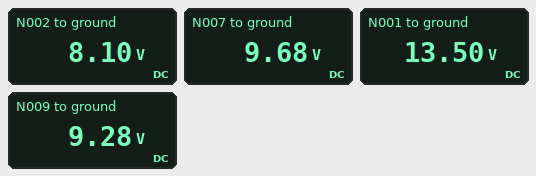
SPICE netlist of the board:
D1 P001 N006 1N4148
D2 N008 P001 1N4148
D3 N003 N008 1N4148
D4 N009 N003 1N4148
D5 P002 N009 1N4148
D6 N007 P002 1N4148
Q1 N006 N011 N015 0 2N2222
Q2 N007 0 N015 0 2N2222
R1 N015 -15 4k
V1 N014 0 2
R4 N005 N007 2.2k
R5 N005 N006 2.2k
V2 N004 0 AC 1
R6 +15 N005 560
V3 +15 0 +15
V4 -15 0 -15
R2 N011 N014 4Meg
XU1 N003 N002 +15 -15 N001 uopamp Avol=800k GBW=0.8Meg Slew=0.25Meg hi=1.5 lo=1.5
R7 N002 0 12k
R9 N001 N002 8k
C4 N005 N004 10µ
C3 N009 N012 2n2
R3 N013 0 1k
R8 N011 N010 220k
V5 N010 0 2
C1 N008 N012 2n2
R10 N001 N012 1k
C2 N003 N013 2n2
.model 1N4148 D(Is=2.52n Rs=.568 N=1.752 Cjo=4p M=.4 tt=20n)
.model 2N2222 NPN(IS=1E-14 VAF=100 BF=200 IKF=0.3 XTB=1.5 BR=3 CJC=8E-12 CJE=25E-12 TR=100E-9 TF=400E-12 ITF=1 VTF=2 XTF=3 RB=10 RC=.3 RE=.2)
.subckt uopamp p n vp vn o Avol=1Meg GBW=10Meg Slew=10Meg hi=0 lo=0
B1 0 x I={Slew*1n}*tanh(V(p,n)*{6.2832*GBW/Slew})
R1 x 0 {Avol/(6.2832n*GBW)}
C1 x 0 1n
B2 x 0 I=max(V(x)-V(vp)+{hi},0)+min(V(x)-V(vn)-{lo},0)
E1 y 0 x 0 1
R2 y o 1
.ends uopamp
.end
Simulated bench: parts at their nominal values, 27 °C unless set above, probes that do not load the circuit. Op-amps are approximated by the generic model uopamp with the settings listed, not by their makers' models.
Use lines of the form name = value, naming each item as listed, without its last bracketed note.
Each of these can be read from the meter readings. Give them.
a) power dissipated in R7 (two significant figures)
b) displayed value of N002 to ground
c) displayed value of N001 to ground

power dissipated in R7 = 5.5 mW
displayed value of N002 to ground = 8.10 V
displayed value of N001 to ground = 13.50 V
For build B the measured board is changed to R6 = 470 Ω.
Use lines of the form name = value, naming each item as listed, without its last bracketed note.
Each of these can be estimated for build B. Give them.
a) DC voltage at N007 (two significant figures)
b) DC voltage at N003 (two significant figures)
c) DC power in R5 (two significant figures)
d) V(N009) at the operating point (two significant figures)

DC voltage at N007 = 10 V
DC voltage at N003 = 9.4 V
DC power in R5 = 9.4 mW
V(N009) at the operating point = 9.6 V
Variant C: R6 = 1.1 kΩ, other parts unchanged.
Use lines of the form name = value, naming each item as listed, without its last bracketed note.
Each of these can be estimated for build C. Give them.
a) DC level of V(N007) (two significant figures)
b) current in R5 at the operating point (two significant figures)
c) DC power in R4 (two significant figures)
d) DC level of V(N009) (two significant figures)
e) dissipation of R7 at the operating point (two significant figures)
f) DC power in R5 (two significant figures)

DC level of V(N007) = 7.7 V
current in R5 at the operating point = 2.0 mA
DC power in R4 = 5.2 mW
DC level of V(N009) = 7.3 V
dissipation of R7 at the operating point = 4.3 mW
DC power in R5 = 9.0 mW
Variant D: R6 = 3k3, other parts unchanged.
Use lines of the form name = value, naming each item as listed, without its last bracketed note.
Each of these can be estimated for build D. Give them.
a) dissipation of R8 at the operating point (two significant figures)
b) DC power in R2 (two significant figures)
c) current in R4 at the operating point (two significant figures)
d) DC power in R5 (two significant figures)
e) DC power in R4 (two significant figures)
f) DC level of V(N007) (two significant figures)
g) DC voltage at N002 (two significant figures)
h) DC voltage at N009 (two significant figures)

dissipation of R8 at the operating point = 18 µW
DC power in R2 = 1.0 µW
current in R4 at the operating point = 1.8 mA
DC power in R5 = 6.7 mW
DC power in R4 = 7.0 mW
DC level of V(N007) = -590 mV
DC voltage at N002 = -550 mV
DC voltage at N009 = -560 mV
